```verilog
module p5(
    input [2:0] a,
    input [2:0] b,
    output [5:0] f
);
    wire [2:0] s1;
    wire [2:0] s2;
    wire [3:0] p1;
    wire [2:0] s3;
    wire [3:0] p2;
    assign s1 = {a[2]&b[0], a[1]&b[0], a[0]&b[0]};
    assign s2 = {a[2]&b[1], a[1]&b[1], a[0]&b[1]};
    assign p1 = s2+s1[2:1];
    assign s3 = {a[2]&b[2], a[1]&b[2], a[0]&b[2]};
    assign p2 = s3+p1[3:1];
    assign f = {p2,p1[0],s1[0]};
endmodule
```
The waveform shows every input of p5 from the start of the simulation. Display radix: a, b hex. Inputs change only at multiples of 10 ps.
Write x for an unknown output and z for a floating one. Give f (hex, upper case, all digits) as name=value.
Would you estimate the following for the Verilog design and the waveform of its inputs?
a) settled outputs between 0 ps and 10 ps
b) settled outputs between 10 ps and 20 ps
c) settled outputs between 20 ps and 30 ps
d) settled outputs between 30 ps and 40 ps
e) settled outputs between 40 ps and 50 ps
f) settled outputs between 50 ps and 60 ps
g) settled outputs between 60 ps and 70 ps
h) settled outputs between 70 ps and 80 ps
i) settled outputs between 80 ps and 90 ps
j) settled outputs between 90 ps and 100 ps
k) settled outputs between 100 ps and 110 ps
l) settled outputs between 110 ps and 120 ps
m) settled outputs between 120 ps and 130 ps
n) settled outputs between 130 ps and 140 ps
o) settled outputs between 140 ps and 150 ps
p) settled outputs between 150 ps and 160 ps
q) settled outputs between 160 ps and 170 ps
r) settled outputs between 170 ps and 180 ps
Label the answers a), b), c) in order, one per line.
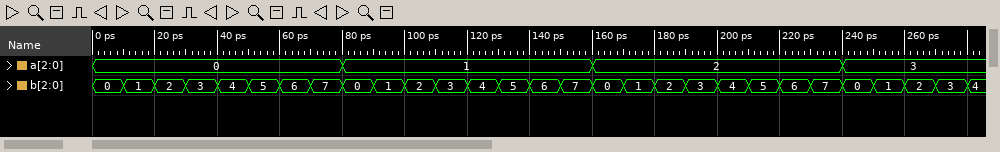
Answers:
a) f=00
b) f=00
c) f=00
d) f=00
e) f=00
f) f=00
g) f=00
h) f=00
i) f=00
j) f=01
k) f=02
l) f=03
m) f=04
n) f=05
o) f=06
p) f=07
q) f=00
r) f=02
